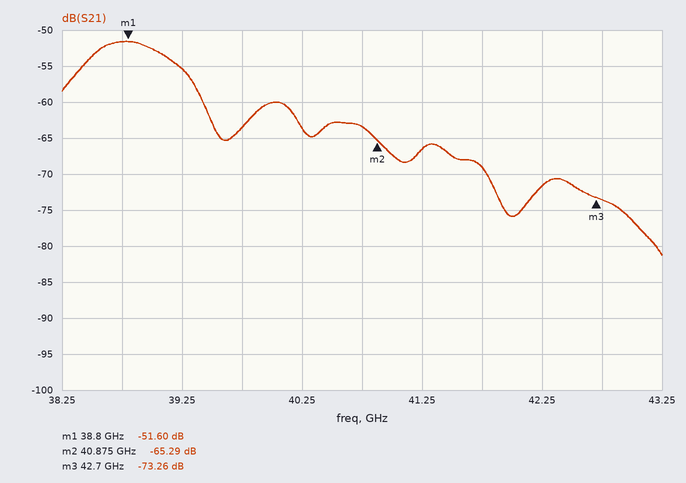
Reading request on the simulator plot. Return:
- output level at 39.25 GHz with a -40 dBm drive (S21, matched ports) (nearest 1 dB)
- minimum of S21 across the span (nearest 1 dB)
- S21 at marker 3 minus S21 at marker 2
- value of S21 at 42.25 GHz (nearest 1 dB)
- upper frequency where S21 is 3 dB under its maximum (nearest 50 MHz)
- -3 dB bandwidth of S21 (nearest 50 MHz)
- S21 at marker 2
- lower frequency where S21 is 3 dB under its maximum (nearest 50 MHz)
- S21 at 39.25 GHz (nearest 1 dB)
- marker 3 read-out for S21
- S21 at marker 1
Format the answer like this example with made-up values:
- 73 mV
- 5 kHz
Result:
- -95 dBm
- -81 dB
- -7.97 dB
- -72 dB
- 39.20 GHz
- 750 MHz
- -65.29 dB
- 38.45 GHz
- -55 dB
- -73.26 dB
- -51.60 dB
